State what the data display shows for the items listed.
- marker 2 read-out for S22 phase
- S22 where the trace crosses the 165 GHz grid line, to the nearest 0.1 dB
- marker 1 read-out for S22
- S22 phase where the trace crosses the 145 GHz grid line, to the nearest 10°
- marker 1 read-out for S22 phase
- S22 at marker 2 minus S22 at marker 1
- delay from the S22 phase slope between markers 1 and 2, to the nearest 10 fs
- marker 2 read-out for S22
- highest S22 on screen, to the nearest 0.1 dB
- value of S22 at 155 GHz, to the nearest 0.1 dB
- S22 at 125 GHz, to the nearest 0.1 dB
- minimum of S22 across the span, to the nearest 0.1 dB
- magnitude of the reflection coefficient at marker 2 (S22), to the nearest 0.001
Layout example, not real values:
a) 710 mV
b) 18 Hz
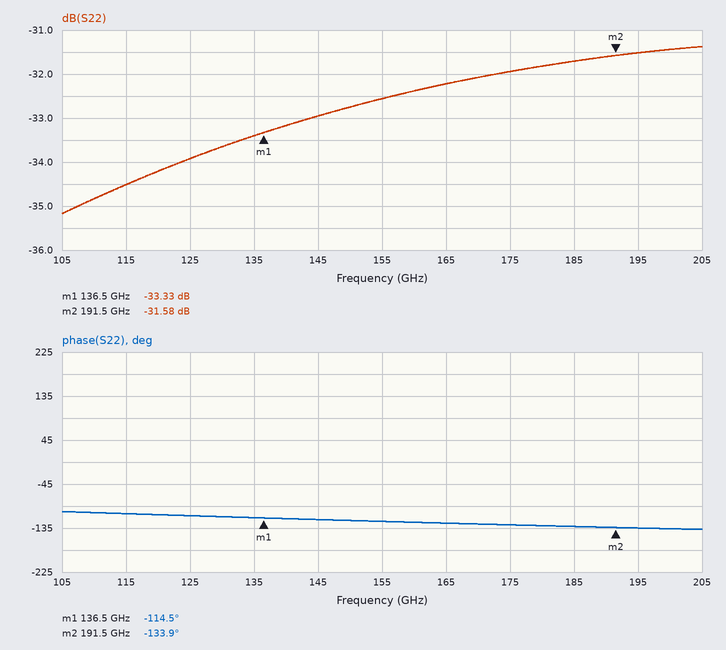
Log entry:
a) -133.9°
b) -32.2 dB
c) -33.33 dB
d) -120°
e) -114.5°
f) 1.75 dB
g) 980 fs
h) -31.58 dB
i) -31.4 dB
j) -32.6 dB
k) -33.9 dB
l) -35.2 dB
m) 0.026
